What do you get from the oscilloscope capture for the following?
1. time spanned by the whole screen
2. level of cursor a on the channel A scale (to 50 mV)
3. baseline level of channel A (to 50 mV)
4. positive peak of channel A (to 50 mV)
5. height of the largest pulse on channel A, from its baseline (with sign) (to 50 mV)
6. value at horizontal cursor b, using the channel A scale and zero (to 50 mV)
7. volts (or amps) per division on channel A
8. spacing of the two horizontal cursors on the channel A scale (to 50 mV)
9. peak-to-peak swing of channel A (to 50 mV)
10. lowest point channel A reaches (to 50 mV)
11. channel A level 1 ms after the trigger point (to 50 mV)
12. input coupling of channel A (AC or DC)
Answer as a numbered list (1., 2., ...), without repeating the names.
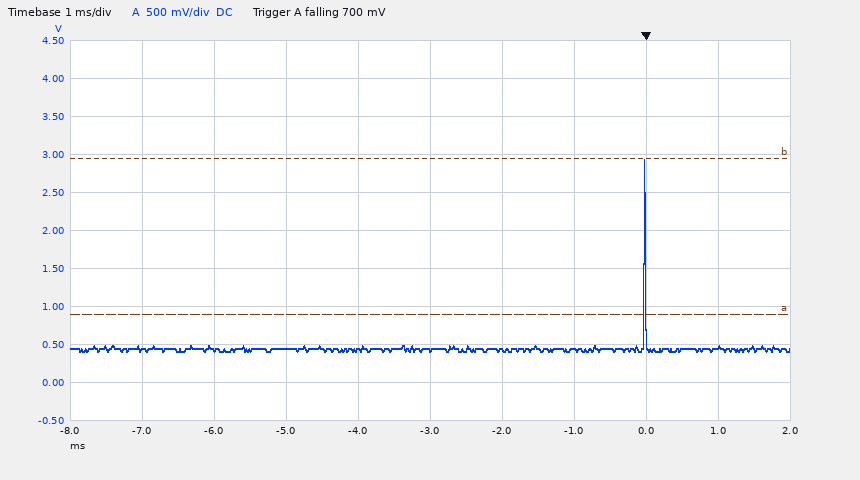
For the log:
1. 10 ms
2. 900 mV
3. 450 mV
4. 2.95 V
5. +2.50 V
6. 2.95 V
7. 500 mV
8. 2.05 V
9. 2.55 V
10. 400 mV
11. 450 mV
12. DC
